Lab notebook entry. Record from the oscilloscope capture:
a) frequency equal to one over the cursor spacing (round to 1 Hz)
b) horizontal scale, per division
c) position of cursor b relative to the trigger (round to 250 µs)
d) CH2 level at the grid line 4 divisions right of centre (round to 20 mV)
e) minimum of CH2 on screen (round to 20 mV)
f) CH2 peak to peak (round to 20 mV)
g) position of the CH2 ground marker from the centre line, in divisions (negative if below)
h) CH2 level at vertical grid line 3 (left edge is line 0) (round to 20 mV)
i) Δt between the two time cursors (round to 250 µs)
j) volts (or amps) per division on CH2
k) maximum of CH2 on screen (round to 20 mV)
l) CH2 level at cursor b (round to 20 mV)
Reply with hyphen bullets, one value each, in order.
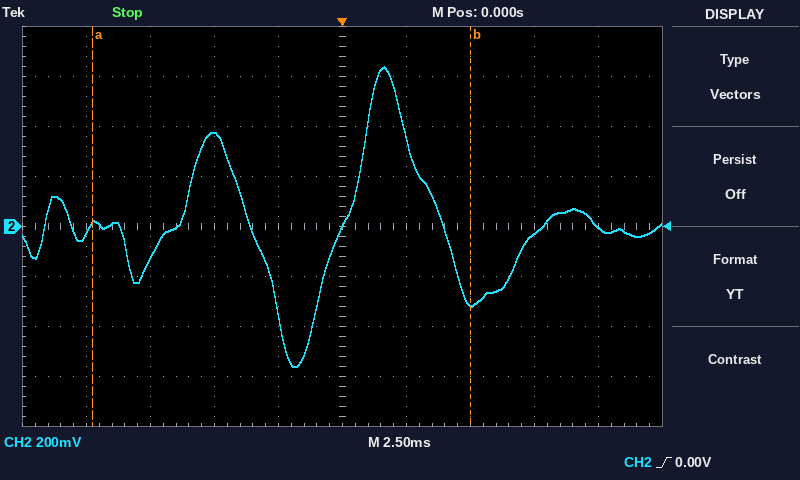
- 68 Hz
- 2.5 ms
- +5.00 ms
- 0 mV
- -560 mV
- 1.20 V
- 0.0 div
- 380 mV
- 14.75 ms
- 200 mV
- 640 mV
- -320 mV
